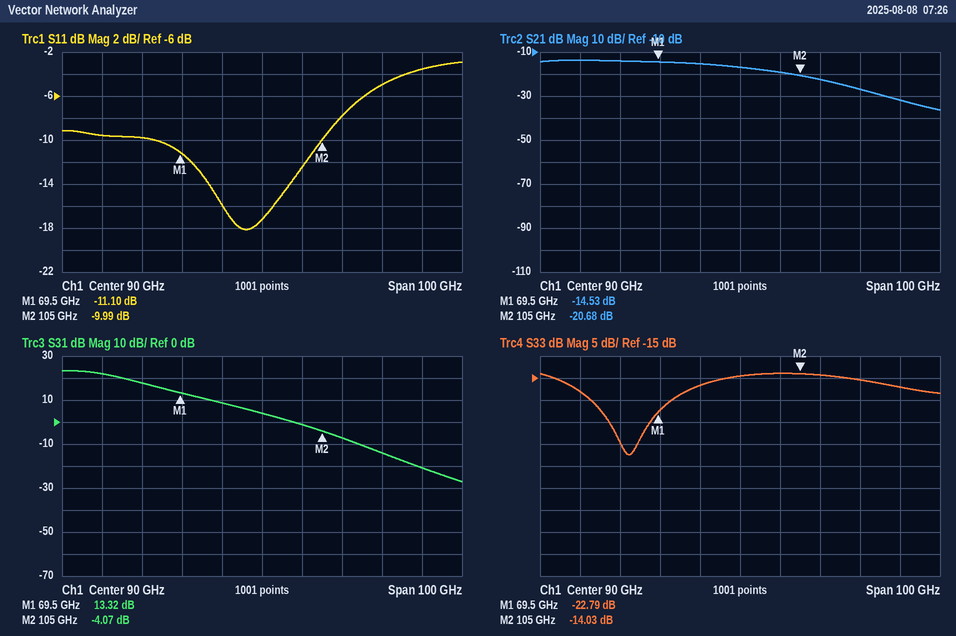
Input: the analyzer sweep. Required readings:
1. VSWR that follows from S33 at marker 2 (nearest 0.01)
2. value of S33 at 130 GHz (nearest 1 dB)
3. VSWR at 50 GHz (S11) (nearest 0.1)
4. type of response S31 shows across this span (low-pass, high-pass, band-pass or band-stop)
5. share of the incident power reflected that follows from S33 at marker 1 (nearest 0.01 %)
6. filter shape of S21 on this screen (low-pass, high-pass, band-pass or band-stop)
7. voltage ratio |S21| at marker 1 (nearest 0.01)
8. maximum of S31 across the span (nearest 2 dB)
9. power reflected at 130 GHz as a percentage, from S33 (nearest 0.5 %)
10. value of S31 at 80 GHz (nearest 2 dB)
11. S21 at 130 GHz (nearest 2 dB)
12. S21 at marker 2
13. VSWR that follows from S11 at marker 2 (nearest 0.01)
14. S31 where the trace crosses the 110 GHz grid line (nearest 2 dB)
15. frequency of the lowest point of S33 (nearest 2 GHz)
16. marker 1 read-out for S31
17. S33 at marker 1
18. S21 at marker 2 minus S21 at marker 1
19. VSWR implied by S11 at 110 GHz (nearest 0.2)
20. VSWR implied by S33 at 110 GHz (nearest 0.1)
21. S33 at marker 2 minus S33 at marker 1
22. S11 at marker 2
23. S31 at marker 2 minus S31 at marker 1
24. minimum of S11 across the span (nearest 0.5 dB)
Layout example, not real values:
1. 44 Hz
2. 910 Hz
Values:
1. 1.50
2. -17 dB
3. 2.0
4. low-pass
5. 0.53 %
6. low-pass
7. 0.19
8. 24 dB
9. 2.0 %
10. 8 dB
11. -32 dB
12. -20.68 dB
13. 1.93
14. -8 dB
15. 62 GHz
16. 13.32 dB
17. -22.79 dB
18. -6.15 dB
19. 2.4
20. 1.5
21. 8.76 dB
22. -9.99 dB
23. -17.39 dB
24. -18.0 dB
